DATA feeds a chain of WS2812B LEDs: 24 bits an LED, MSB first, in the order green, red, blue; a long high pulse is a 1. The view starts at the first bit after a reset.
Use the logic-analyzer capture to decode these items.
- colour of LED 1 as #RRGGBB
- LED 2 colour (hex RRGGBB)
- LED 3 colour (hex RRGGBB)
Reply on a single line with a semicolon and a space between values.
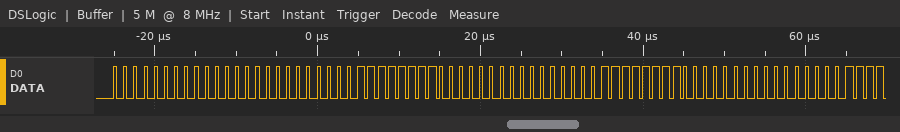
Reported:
#000000; #00FF00; #00FF00
